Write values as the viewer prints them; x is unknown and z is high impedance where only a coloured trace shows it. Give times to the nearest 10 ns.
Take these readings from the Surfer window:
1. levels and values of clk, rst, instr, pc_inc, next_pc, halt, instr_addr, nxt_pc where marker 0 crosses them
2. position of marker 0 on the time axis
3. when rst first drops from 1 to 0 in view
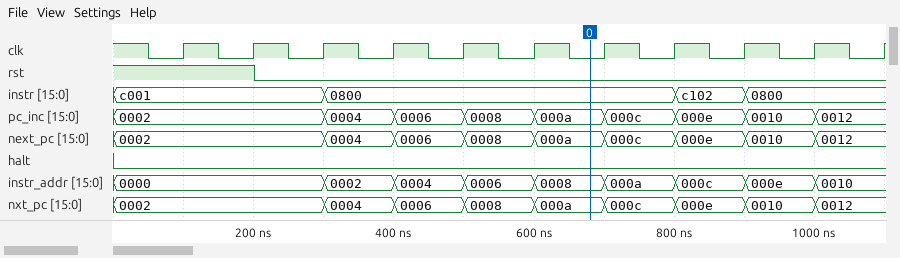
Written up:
clk=0, rst=0, instr=0800, pc_inc=000a, next_pc=000a, halt=0, instr_addr=0008, nxt_pc=000a
680 ns
200 ns
